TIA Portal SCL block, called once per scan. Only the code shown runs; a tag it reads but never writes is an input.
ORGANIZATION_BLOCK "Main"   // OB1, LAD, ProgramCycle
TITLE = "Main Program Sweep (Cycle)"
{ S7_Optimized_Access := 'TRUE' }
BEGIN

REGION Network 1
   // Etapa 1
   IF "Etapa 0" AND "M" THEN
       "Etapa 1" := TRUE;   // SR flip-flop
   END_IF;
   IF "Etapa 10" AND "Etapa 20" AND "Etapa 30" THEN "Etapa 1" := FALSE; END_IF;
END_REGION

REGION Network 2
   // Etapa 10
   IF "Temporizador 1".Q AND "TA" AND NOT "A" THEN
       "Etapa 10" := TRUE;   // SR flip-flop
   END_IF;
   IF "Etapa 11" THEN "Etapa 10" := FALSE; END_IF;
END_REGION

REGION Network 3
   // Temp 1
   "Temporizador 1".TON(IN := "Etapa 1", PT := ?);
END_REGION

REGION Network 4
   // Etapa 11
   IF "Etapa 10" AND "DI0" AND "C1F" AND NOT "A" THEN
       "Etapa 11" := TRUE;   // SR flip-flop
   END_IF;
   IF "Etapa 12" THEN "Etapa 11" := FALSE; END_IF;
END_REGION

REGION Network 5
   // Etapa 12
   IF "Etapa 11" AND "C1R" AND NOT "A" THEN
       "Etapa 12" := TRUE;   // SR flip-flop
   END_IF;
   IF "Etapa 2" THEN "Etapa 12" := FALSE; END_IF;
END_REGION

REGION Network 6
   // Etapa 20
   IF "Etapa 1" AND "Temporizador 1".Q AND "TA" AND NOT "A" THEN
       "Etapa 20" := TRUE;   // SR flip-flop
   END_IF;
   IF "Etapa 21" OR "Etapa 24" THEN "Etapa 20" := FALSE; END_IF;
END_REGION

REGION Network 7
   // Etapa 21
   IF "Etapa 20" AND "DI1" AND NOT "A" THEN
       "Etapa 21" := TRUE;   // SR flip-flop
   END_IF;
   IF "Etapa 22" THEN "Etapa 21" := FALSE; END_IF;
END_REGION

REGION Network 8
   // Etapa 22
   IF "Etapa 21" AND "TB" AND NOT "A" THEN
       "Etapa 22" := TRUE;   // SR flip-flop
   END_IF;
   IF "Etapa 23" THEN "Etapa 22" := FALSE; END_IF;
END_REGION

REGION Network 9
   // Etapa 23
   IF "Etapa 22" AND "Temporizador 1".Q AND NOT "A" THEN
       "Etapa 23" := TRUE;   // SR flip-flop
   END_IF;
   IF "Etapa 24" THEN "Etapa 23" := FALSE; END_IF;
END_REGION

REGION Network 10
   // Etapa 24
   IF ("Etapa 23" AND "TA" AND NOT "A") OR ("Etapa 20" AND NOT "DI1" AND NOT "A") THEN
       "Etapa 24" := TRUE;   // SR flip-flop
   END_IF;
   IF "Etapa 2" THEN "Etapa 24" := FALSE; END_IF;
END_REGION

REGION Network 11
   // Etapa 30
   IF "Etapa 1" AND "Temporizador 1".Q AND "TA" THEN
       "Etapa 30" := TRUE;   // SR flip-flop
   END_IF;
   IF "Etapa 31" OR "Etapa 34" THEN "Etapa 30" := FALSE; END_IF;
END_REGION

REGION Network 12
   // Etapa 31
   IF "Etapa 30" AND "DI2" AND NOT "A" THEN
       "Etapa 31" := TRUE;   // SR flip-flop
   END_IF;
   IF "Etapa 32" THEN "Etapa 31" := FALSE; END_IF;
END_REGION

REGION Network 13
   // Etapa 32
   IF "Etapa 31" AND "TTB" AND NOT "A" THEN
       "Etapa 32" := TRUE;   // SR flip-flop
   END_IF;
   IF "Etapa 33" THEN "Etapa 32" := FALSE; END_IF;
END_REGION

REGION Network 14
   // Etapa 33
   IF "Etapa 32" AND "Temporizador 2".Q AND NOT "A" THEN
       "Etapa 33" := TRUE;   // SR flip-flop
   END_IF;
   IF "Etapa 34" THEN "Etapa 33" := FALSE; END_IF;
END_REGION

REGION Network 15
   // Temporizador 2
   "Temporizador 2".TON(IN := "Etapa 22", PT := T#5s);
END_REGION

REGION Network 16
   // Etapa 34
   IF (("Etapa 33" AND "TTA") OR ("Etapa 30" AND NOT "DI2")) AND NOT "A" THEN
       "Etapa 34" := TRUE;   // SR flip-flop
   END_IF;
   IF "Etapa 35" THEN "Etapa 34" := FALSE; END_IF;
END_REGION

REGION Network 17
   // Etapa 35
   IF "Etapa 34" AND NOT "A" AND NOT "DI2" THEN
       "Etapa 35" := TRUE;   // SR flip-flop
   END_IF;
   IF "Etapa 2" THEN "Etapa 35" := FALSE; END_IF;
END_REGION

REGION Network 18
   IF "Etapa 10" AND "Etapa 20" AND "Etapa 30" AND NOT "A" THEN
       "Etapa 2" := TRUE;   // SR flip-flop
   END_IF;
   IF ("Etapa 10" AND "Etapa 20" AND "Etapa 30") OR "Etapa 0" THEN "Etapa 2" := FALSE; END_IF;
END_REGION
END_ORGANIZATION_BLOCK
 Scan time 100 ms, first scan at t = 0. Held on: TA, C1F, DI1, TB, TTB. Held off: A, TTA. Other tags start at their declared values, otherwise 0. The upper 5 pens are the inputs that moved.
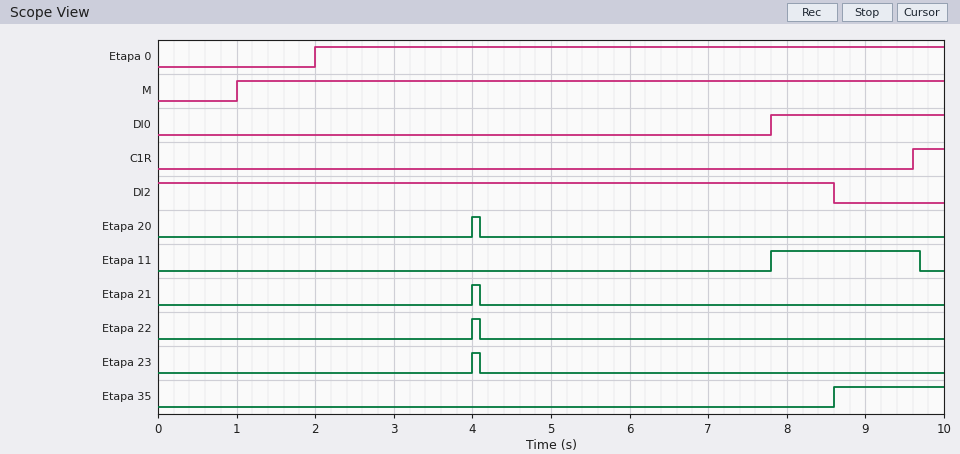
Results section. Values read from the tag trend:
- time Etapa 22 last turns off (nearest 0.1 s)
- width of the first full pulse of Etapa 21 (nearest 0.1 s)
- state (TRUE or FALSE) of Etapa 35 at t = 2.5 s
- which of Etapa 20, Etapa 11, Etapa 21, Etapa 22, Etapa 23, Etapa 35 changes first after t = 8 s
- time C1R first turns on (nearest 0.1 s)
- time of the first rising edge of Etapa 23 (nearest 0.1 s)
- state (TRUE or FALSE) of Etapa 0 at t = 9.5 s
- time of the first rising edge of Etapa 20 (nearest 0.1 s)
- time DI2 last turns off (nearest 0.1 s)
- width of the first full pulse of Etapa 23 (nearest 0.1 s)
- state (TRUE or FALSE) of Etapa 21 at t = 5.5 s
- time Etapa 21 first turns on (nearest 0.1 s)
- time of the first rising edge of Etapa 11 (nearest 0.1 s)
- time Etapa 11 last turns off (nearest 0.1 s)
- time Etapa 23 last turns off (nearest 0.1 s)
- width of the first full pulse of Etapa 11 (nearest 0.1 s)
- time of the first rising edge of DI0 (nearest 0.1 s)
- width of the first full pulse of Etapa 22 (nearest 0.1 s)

4.1 s
0.1 s
FALSE
Etapa 35
9.6 s
4.0 s
TRUE
4.0 s
8.6 s
0.1 s
FALSE
4.0 s
7.8 s
9.7 s
4.1 s
1.9 s
7.8 s
0.1 s
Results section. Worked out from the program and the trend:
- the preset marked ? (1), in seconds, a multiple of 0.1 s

2.0 s
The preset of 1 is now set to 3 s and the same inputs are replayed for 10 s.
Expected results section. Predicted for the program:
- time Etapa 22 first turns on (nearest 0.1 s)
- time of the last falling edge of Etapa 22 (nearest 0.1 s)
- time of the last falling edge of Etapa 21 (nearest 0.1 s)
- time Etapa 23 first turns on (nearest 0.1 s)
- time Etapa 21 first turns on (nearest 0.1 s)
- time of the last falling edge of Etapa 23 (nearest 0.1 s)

5.0 s
5.1 s
5.1 s
5.0 s
5.0 s
5.1 s
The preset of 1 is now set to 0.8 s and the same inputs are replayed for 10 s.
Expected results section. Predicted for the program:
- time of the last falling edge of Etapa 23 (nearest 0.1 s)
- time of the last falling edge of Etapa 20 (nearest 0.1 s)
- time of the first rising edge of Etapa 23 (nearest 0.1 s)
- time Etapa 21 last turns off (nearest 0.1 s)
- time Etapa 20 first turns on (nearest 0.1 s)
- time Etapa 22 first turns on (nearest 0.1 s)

2.9 s
2.9 s
2.8 s
2.9 s
2.8 s
2.8 s
